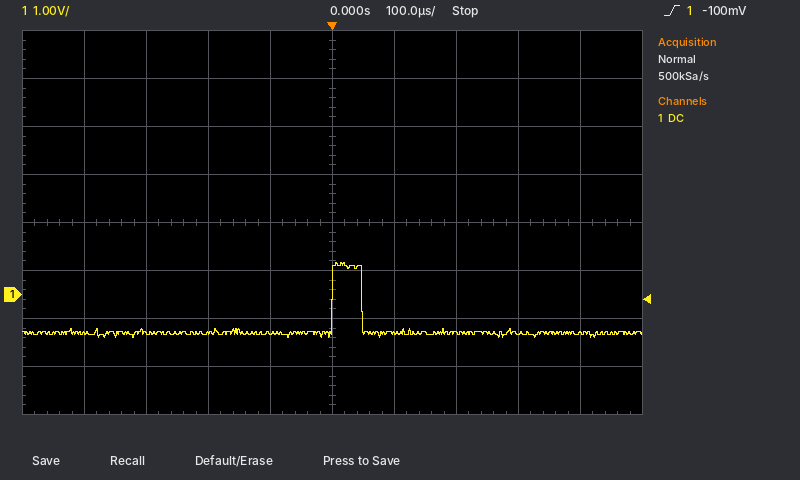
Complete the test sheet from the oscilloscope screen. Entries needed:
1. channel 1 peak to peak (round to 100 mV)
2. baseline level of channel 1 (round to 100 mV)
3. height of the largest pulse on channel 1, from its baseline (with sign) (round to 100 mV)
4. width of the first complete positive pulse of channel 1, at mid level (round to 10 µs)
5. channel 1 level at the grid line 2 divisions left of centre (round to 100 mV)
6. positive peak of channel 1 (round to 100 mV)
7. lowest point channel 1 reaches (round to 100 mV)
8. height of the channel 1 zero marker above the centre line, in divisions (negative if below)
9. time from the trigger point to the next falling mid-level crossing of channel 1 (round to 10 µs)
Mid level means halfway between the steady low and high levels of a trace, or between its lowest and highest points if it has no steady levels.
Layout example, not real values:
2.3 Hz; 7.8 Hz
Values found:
1.6 V; -800 mV; +1.5 V; 50 µs; -800 mV; 700 mV; -900 mV; -1.5 div; 50 µs
